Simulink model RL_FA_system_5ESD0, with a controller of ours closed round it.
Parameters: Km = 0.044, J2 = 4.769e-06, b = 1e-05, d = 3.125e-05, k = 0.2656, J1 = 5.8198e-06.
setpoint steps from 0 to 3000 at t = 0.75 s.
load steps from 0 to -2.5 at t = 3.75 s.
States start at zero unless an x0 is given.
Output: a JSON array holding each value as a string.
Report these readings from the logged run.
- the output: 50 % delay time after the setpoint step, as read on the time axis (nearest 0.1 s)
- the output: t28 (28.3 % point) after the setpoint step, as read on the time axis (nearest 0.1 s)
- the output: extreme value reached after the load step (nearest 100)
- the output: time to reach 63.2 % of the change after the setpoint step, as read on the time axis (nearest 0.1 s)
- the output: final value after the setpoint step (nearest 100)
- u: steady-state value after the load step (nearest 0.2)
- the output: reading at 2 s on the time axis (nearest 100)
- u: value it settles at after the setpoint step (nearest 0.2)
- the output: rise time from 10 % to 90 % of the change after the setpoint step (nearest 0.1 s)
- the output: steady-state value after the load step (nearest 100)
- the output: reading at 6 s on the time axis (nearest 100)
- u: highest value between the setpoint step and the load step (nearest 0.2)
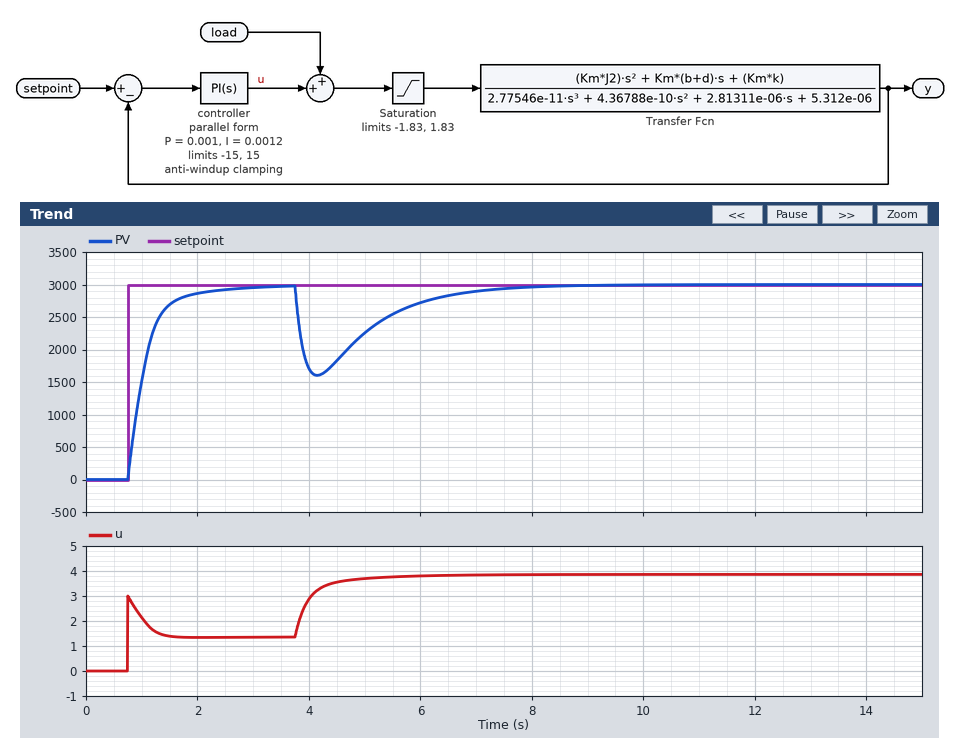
["1.0 s", "0.9 s", "1600", "1.1 s", "3000", "3.8", "2900", "1.4", "0.7 s", "3000", "2700", "3.0"]
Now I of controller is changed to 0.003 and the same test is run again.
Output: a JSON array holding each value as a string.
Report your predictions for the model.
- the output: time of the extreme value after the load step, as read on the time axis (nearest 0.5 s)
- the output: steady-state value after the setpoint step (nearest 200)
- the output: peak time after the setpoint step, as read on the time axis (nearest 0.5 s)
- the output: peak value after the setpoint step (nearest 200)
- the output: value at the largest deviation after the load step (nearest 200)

["4.0 s", "3000", "2.0 s", "3600", "1800"]
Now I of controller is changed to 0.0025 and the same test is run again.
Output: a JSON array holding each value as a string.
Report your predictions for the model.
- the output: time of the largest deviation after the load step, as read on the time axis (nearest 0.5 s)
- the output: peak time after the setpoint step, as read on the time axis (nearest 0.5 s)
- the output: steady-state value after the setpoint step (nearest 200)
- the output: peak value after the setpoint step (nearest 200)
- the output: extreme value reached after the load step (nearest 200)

["4.0 s", "2.0 s", "3000", "3400", "1800"]
